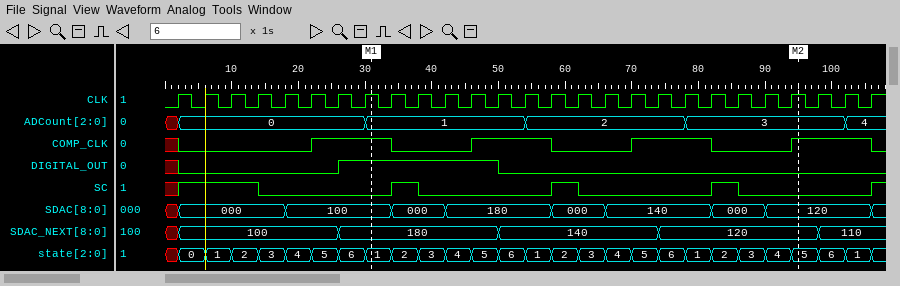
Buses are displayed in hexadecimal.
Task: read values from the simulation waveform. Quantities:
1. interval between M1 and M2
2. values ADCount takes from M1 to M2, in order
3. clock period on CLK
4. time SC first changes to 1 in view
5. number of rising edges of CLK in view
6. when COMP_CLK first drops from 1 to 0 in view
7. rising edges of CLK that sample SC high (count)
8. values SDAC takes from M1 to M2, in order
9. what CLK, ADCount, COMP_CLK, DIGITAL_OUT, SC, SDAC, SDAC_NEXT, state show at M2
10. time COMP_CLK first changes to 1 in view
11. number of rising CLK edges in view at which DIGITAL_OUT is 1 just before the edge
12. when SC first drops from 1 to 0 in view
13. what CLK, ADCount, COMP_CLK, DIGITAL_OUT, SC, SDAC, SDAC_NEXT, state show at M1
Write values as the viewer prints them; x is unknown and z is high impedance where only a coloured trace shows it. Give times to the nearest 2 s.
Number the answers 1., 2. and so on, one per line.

1. 64 s
2. 1, 2, 3
3. 4 s
4. 2 s
5. 27
6. 34 s
7. 6
8. 100, 000, 180, 000, 140, 000, 120
9. CLK=1, ADCount=3, COMP_CLK=1, DIGITAL_OUT=0, SC=0, SDAC=120, SDAC_NEXT=120, state=5
10. 22 s
11. 6
12. 14 s
13. CLK=1, ADCount=1, COMP_CLK=1, DIGITAL_OUT=1, SC=0, SDAC=100, SDAC_NEXT=180, state=1
